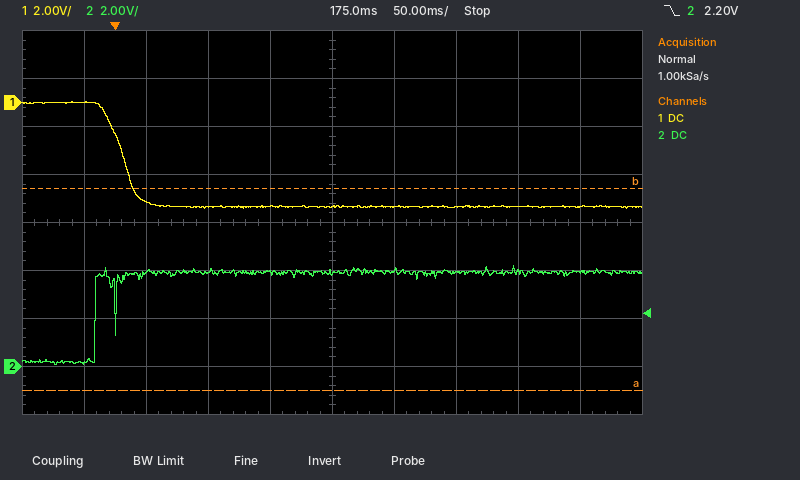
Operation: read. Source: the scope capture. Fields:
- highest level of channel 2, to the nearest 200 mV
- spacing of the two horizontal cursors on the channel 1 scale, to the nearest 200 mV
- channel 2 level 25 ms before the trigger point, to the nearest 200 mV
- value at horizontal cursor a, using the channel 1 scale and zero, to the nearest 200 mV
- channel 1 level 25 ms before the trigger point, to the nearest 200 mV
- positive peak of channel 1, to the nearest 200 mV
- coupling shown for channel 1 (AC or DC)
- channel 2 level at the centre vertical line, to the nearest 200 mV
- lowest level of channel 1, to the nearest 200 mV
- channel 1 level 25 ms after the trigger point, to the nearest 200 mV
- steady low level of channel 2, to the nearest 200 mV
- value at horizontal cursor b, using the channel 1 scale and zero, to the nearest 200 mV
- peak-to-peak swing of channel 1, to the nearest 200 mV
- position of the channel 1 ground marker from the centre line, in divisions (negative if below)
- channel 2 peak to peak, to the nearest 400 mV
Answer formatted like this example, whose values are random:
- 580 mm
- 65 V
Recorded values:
- 4.2 V
- 8.4 V
- 200 mV
- -12.0 V
- 0.0 V
- 0.0 V
- DC
- 4.0 V
- -4.4 V
- -4.2 V
- 200 mV
- -3.6 V
- 4.4 V
- +2.5 div
- 4.0 V
